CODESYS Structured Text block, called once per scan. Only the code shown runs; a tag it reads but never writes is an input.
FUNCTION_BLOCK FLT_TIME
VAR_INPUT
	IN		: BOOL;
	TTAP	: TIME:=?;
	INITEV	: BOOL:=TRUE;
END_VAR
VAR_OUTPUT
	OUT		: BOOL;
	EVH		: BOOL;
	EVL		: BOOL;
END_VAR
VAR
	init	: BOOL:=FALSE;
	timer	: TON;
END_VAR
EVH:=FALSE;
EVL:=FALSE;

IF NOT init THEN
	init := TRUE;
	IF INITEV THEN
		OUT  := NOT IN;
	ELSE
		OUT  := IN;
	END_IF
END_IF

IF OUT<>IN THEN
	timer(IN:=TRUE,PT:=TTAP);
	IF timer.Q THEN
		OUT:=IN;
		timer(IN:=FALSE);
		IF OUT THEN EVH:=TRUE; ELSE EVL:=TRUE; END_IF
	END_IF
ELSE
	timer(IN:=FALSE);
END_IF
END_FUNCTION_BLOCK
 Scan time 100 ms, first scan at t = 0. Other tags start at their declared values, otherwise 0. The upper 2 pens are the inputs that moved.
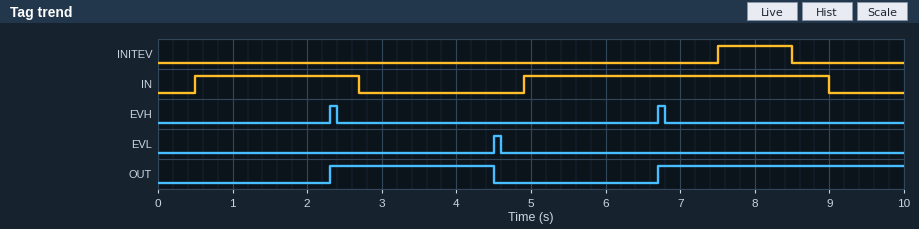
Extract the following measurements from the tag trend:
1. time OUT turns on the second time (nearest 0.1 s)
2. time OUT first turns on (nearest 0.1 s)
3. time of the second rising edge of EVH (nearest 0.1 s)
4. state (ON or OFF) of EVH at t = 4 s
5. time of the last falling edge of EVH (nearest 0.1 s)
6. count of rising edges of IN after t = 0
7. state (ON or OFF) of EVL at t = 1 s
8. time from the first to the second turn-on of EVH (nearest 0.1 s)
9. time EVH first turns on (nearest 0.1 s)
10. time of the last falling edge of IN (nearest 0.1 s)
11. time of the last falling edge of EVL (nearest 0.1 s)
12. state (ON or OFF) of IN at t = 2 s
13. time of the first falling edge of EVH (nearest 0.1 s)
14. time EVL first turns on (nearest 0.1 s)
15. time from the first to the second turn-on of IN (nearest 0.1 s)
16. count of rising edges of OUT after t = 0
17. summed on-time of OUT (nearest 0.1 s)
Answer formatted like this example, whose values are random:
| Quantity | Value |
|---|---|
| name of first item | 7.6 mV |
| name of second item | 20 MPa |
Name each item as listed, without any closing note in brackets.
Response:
| Quantity | Value |
|---|---|
| time OUT turns on the second time | 6.7 s |
| time OUT first turns on | 2.3 s |
| time of the second rising edge of EVH | 6.7 s |
| state (ON or OFF) of EVH at t = 4 s | OFF |
| time of the last falling edge of EVH | 6.8 s |
| count of rising edges of IN after t = 0 | 2 |
| state (ON or OFF) of EVL at t = 1 s | OFF |
| time from the first to the second turn-on of EVH | 4.4 s |
| time EVH first turns on | 2.3 s |
| time of the last falling edge of IN | 9.0 s |
| time of the last falling edge of EVL | 4.6 s |
| state (ON or OFF) of IN at t = 2 s | ON |
| time of the first falling edge of EVH | 2.4 s |
| time EVL first turns on | 4.5 s |
| time from the first to the second turn-on of IN | 4.4 s |
| count of rising edges of OUT after t = 0 | 2 |
| summed on-time of OUT | 5.5 s |
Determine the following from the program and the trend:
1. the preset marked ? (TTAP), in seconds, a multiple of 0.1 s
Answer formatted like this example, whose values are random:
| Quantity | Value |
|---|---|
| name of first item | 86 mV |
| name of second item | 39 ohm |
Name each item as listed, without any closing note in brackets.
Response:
| Quantity | Value |
|---|---|
| the preset marked ? (TTAP), in seconds, a multiple of 0.1 s | 1.8 s |
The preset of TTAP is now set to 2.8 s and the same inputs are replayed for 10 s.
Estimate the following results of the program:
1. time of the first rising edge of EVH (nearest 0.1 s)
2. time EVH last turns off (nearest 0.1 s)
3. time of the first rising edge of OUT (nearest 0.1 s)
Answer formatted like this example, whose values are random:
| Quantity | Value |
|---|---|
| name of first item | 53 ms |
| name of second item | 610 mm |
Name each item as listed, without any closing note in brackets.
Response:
| Quantity | Value |
|---|---|
| time of the first rising edge of EVH | 7.7 s |
| time EVH last turns off | 7.8 s |
| time of the first rising edge of OUT | 7.7 s |
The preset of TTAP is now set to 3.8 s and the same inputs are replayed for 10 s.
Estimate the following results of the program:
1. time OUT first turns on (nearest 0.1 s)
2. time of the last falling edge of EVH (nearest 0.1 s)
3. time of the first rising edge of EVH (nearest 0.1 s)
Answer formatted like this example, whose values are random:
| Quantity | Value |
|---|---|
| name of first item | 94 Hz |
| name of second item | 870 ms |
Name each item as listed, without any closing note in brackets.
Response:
| Quantity | Value |
|---|---|
| time OUT first turns on | 8.7 s |
| time of the last falling edge of EVH | 8.8 s |
| time of the first rising edge of EVH | 8.7 s |
